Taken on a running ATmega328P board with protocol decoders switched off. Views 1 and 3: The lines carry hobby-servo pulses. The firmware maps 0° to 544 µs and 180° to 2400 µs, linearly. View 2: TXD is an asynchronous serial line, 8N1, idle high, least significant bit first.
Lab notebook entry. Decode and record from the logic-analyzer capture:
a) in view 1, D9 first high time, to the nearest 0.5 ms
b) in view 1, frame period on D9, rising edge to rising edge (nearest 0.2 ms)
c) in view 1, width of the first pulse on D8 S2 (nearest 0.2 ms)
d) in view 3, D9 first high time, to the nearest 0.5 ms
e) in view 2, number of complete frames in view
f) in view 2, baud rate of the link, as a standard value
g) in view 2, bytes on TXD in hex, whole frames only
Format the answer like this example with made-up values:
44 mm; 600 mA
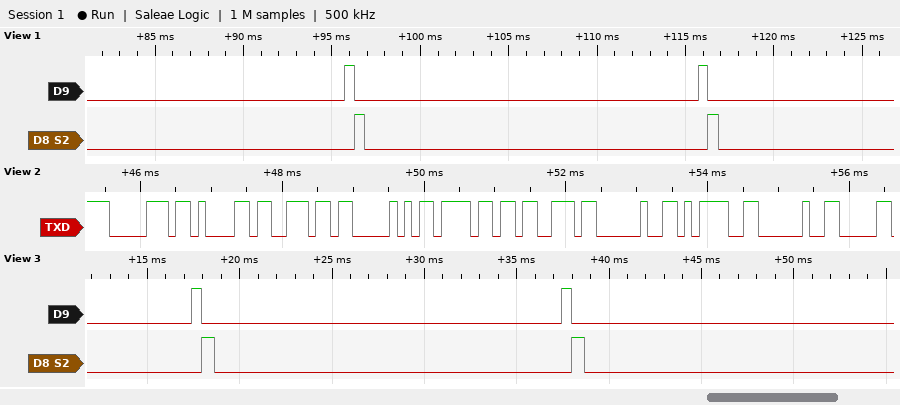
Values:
0.5 ms; 20.0 ms; 0.6 ms; 0.5 ms; 9; 9600 baud; 70 61 6E 50 6F 73 20 3D 20
